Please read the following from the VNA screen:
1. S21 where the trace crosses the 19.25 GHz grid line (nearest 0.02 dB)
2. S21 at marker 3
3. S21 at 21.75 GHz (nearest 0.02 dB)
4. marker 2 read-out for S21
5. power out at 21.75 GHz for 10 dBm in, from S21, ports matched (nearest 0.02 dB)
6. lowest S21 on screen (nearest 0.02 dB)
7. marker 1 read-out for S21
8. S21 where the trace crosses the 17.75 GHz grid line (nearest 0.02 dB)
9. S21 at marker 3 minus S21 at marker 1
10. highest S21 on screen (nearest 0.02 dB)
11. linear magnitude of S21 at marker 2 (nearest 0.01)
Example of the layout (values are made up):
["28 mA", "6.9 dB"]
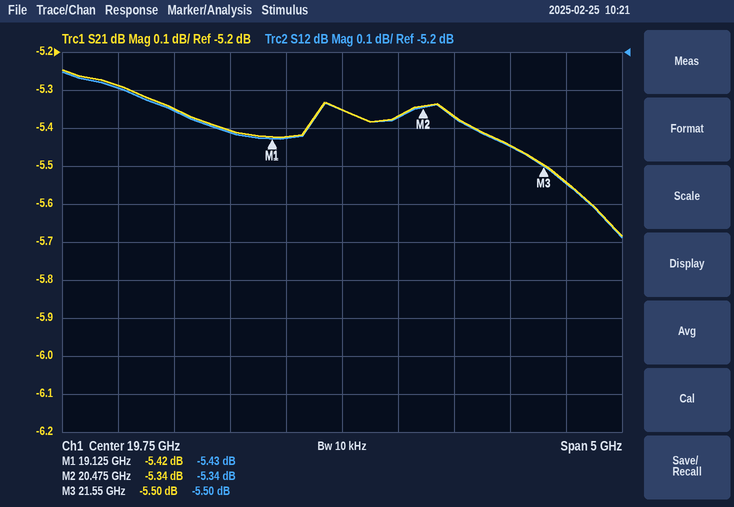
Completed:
["-5.42 dB", "-5.50 dB", "-5.54 dB", "-5.34 dB", "4.46 dBm", "-5.68 dB", "-5.42 dB", "-5.28 dB", "-0.08 dB", "-5.24 dB", "0.54"]
